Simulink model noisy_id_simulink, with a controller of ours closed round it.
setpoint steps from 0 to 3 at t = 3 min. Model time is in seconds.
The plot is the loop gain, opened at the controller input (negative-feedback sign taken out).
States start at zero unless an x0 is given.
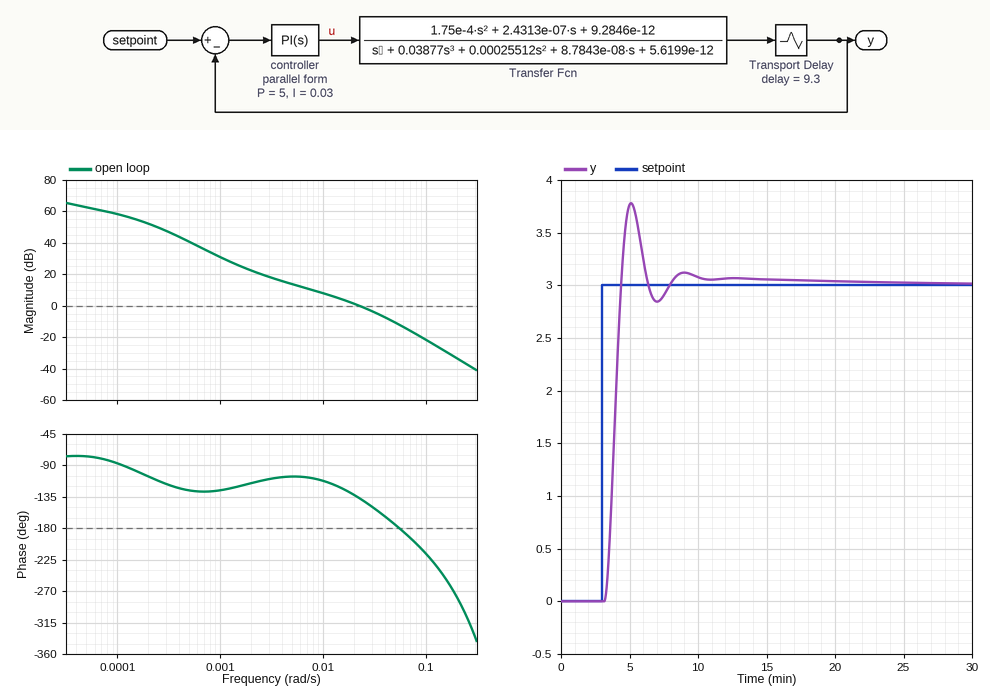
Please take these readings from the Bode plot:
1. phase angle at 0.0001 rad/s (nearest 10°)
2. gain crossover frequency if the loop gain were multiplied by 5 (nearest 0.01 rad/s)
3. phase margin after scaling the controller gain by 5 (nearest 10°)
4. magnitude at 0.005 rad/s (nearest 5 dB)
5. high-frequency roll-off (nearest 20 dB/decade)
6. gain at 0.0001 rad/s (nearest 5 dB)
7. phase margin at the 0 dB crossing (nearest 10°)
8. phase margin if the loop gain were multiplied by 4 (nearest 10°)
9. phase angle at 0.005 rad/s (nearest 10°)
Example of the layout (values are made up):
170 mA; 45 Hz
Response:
-90°; 0.06 rad/s; -10°; 15 dB; -40 dB/decade; 60 dB; 40°; 0°; -110°
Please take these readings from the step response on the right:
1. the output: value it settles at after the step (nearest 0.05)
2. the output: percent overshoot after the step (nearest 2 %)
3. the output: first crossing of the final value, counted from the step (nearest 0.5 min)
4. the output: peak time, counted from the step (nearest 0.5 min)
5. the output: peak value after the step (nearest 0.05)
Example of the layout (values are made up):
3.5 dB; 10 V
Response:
3.00; 26 %; 1.5 min; 2.0 min; 3.80
